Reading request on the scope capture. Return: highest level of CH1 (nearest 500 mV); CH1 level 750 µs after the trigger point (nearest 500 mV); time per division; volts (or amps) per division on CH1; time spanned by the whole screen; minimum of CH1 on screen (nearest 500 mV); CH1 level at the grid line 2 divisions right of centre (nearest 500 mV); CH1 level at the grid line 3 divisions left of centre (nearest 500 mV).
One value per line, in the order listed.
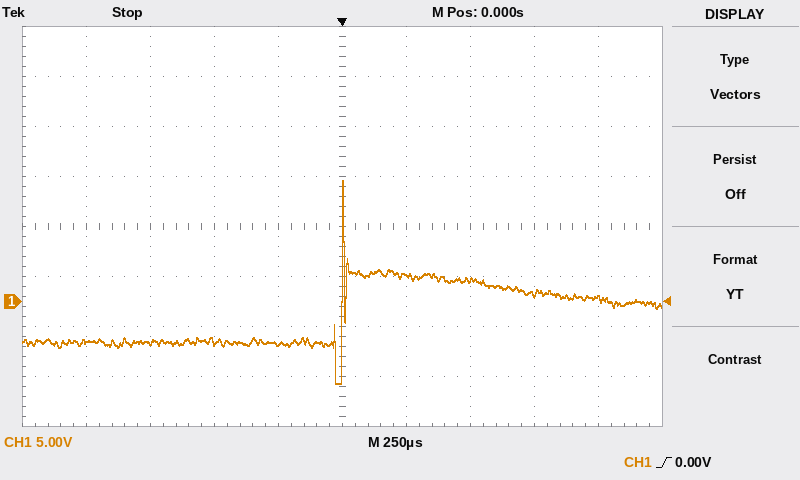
12.0 V
1.0 V
250 µs
5 V
2.5 ms
-8.0 V
2.0 V
-4.0 V
